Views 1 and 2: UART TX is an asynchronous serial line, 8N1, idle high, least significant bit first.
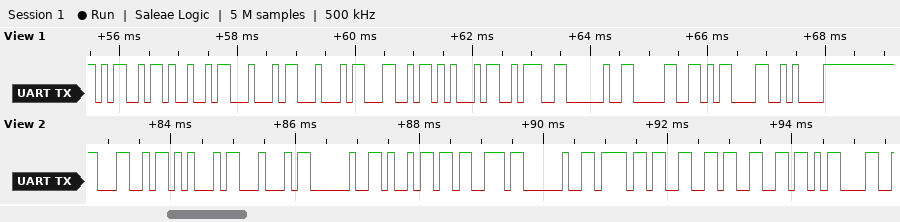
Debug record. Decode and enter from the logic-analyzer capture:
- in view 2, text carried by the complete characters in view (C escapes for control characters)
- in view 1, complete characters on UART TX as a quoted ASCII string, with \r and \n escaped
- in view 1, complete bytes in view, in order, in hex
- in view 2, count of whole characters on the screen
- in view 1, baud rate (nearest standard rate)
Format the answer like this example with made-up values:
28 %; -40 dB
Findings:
"LED is off\r"; "MIDDLE: 0\r\n"; 4D 49 44 44 4C 45 3A 20 30 0D 0A; 11; 9600 baud
